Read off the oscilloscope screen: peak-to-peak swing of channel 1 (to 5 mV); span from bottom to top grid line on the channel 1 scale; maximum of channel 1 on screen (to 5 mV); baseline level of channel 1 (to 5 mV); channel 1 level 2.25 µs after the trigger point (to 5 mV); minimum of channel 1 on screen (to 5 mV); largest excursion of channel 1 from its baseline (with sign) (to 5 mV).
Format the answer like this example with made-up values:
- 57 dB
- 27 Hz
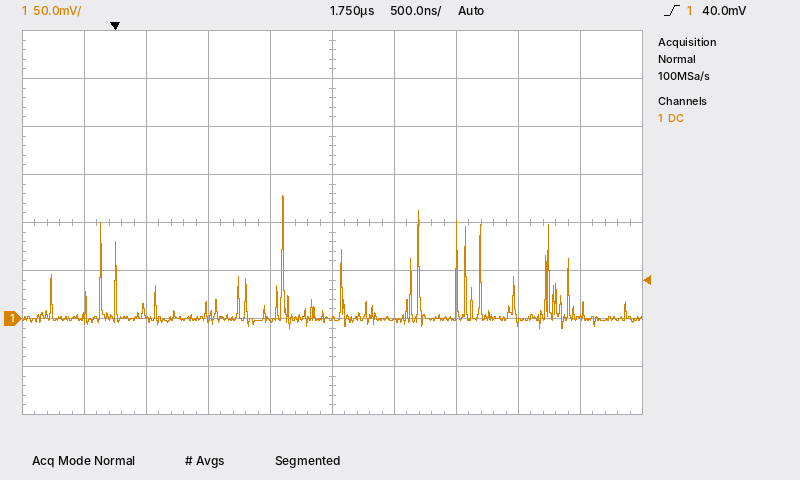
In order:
- 140 mV
- 400 mV
- 130 mV
- 0 mV
- 0 mV
- -10 mV
- +130 mV
